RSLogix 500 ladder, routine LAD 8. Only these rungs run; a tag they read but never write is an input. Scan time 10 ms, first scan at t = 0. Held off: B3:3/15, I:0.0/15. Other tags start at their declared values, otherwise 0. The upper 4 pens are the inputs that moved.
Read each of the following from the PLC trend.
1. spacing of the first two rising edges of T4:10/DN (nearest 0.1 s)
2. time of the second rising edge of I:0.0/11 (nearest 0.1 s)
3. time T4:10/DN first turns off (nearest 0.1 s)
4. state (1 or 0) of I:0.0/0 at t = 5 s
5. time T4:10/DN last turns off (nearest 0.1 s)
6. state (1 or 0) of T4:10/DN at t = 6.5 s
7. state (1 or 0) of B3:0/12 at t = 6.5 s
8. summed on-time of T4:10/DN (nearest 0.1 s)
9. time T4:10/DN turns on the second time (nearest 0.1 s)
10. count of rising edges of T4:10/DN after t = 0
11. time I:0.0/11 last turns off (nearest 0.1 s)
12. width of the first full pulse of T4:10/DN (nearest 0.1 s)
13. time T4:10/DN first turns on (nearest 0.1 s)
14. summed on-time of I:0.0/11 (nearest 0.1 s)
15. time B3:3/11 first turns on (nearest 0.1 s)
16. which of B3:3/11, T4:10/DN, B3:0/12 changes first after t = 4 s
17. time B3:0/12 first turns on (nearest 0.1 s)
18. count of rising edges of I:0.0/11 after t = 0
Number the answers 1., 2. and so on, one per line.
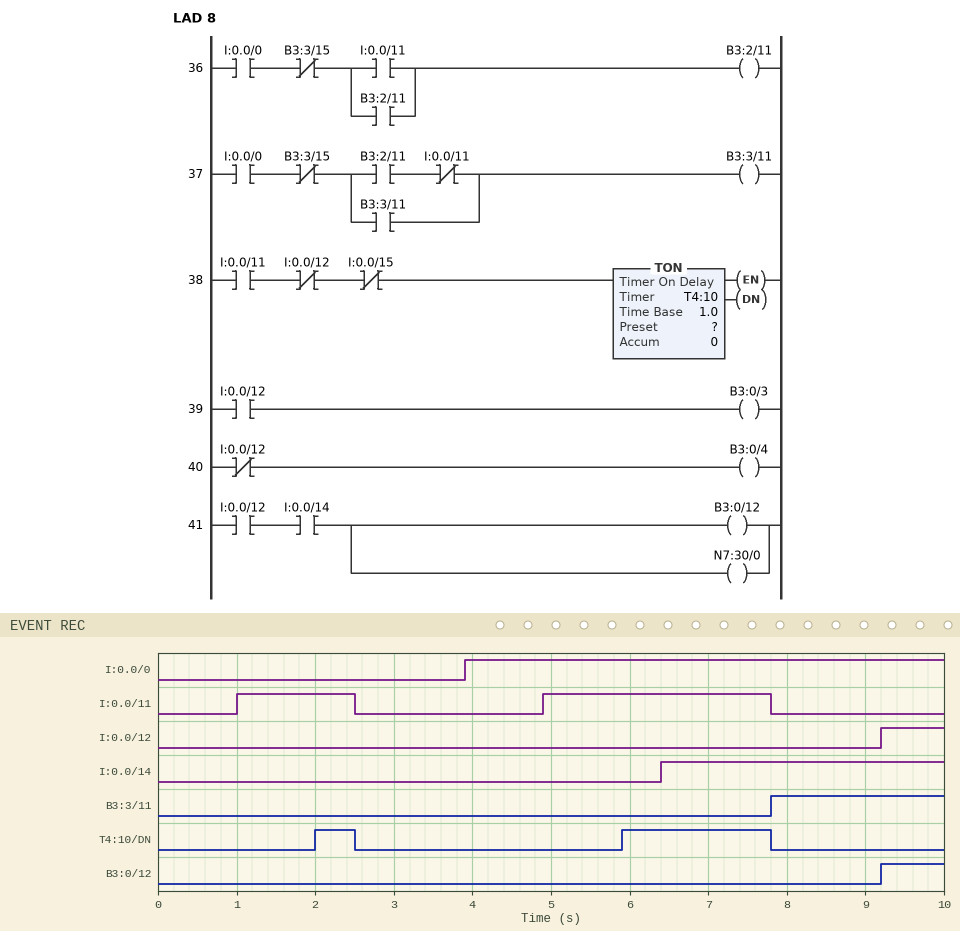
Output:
1. 3.9 s
2. 4.9 s
3. 2.5 s
4. 1
5. 7.8 s
6. 1
7. 0
8. 2.4 s
9. 5.9 s
10. 2
11. 7.8 s
12. 0.5 s
13. 2.0 s
14. 4.4 s
15. 7.8 s
16. T4:10/DN
17. 9.2 s
18. 2
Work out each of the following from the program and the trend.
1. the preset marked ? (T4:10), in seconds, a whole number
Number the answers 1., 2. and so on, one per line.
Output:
1. 1 s
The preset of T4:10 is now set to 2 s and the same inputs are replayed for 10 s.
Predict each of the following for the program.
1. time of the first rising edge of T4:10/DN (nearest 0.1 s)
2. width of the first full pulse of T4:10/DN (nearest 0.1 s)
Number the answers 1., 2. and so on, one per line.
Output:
1. 6.9 s
2. 0.9 s
